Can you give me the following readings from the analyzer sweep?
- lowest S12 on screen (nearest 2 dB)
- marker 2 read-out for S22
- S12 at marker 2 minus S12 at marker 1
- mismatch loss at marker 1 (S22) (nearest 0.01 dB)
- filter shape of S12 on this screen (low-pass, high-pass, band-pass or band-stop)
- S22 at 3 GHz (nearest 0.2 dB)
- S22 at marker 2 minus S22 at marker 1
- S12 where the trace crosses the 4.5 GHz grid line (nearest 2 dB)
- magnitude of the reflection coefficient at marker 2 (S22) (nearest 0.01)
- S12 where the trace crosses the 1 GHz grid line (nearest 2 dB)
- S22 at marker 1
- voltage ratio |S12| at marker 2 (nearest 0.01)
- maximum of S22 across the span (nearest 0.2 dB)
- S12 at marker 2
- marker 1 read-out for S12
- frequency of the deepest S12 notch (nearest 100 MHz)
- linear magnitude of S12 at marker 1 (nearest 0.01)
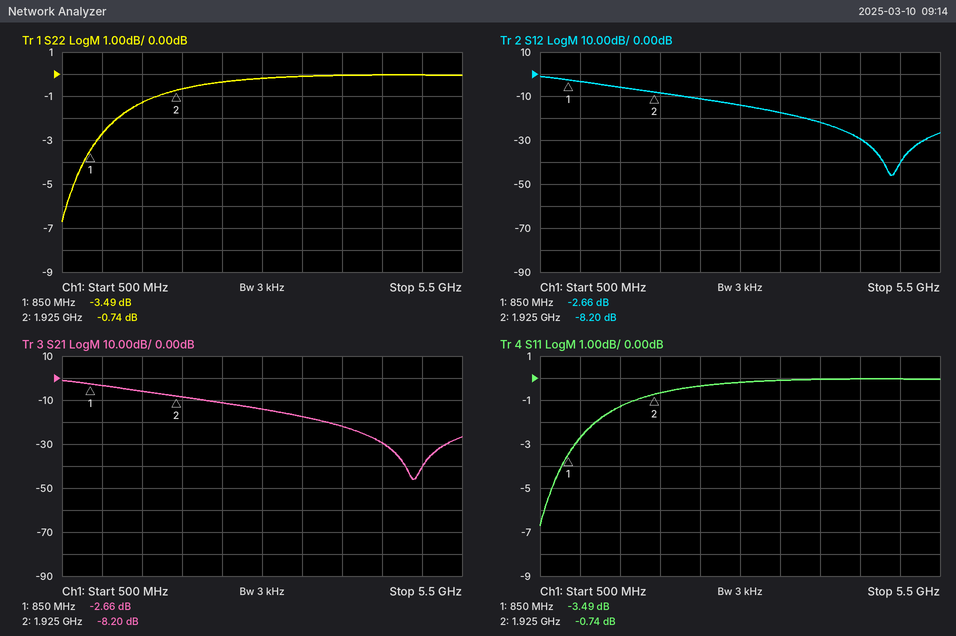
-46 dB
-0.74 dB
-5.54 dB
2.58 dB
low-pass
-0.2 dB
2.75 dB
-30 dB
0.92
-4 dB
-3.49 dB
0.39
0.0 dB
-8.20 dB
-2.66 dB
4.9 GHz
0.74
